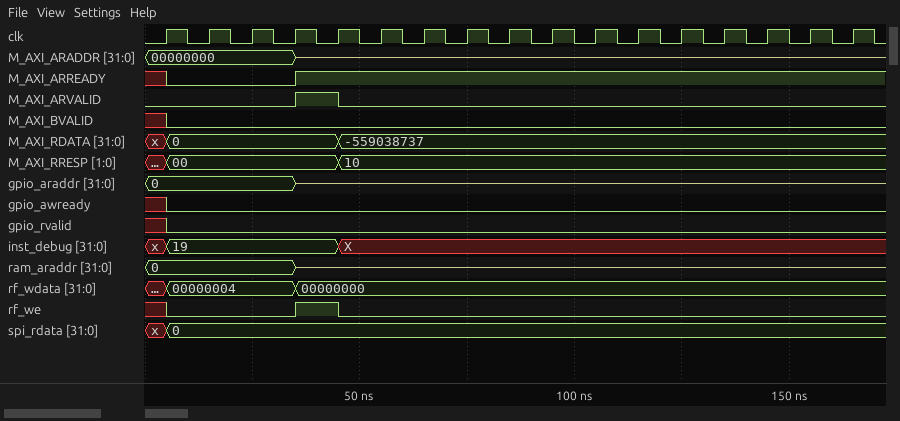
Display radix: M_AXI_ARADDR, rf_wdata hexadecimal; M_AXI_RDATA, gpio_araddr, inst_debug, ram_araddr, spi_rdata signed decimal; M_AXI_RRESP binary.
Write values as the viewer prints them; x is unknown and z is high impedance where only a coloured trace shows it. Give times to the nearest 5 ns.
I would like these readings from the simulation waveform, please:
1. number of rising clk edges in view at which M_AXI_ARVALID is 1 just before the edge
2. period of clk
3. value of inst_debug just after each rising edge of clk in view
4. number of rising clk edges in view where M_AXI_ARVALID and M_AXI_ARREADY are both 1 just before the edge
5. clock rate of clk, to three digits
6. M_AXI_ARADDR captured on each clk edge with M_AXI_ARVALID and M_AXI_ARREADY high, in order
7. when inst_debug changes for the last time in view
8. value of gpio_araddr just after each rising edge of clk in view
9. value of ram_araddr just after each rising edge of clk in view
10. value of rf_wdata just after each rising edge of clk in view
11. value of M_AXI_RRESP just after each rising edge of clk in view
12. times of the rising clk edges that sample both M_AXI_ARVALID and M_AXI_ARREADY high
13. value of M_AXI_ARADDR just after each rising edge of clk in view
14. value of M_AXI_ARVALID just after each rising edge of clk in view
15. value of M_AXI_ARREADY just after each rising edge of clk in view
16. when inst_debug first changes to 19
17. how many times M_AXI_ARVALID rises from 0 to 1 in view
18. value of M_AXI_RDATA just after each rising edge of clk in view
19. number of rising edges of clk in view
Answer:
1
10 ns
19, 19, 19, 19, X, X, X, X, X, X, X, X, X, X, X, X, X
1
100 MHz
z
45 ns
0, 0, 0, z, z, z, z, z, z, z, z, z, z, z, z, z, z
0, 0, 0, z, z, z, z, z, z, z, z, z, z, z, z, z, z
00000004, 00000004, 00000004, 00000000, 00000000, 00000000, 00000000, 00000000, 00000000, 00000000, 00000000, 00000000, 00000000, 00000000, 00000000, 00000000, 00000000
00, 00, 00, 00, 10, 10, 10, 10, 10, 10, 10, 10, 10, 10, 10, 10, 10
45 ns
00000000, 00000000, 00000000, z, z, z, z, z, z, z, z, z, z, z, z, z, z
0 0 0 1 0 0 0 0 0 0 0 0 0 0 0 0 0
0 0 0 1 1 1 1 1 1 1 1 1 1 1 1 1 1
5 ns
1
0, 0, 0, 0, -559038737, -559038737, -559038737, -559038737, -559038737, -559038737, -559038737, -559038737, -559038737, -559038737, -559038737, -559038737, -559038737
17
